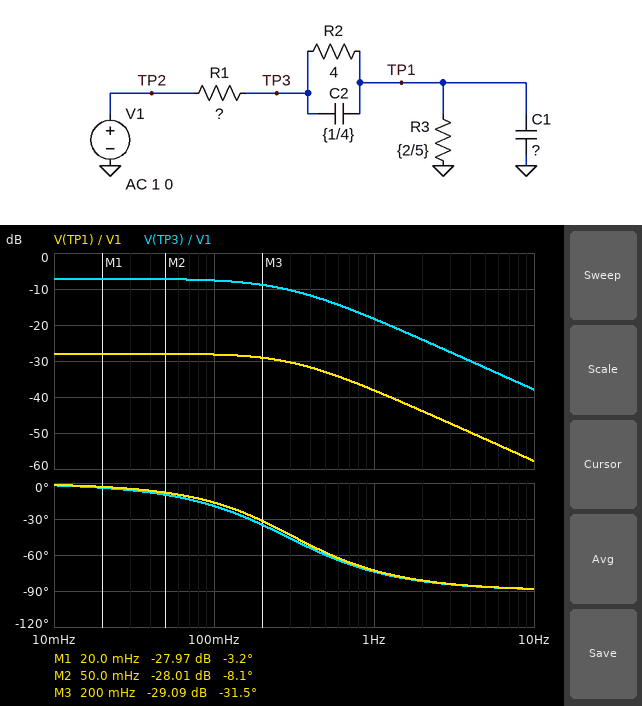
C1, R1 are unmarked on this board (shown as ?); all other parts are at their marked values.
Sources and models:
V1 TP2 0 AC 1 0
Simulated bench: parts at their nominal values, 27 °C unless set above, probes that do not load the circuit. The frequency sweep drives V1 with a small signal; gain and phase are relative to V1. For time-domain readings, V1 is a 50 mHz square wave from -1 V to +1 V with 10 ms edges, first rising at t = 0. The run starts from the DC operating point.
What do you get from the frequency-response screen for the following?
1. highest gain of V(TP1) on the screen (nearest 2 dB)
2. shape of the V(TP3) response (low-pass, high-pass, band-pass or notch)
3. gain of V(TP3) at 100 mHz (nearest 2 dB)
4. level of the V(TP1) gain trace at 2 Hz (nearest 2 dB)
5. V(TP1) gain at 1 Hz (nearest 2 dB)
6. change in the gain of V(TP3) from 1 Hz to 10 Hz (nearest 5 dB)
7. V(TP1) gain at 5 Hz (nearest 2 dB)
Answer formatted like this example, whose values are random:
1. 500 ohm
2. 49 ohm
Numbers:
1. -28 dB
2. low-pass
3. -8 dB
4. -44 dB
5. -38 dB
6. -20 dB
7. -52 dB
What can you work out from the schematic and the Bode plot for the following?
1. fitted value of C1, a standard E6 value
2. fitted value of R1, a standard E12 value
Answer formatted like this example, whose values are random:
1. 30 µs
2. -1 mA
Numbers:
1. 2.2 F
2. 5.6 Ω
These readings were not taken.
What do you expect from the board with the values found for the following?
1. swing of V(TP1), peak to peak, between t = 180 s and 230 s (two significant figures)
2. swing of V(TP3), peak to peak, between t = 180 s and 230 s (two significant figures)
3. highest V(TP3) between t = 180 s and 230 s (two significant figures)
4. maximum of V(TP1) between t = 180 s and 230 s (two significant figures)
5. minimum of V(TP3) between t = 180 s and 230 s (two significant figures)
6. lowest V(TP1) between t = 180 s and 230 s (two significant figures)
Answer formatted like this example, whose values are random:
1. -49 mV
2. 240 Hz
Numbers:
1. 81 mV
2. 880 mV
3. 440 mV
4. 40 mV
5. -440 mV
6. -40 mV
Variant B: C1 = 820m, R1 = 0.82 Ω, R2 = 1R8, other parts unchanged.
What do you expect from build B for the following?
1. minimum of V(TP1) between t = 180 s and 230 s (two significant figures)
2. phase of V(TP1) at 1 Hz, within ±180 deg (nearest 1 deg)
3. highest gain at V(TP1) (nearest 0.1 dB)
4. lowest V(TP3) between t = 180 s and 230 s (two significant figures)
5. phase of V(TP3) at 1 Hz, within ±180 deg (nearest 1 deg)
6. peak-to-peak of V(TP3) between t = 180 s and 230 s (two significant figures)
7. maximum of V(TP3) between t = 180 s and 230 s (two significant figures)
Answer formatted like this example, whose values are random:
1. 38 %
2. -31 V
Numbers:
1. -160 mV
2. -31 deg
3. -16.8 dB
4. -730 mV
5. -36 deg
6. 1.5 V
7. 730 mV
